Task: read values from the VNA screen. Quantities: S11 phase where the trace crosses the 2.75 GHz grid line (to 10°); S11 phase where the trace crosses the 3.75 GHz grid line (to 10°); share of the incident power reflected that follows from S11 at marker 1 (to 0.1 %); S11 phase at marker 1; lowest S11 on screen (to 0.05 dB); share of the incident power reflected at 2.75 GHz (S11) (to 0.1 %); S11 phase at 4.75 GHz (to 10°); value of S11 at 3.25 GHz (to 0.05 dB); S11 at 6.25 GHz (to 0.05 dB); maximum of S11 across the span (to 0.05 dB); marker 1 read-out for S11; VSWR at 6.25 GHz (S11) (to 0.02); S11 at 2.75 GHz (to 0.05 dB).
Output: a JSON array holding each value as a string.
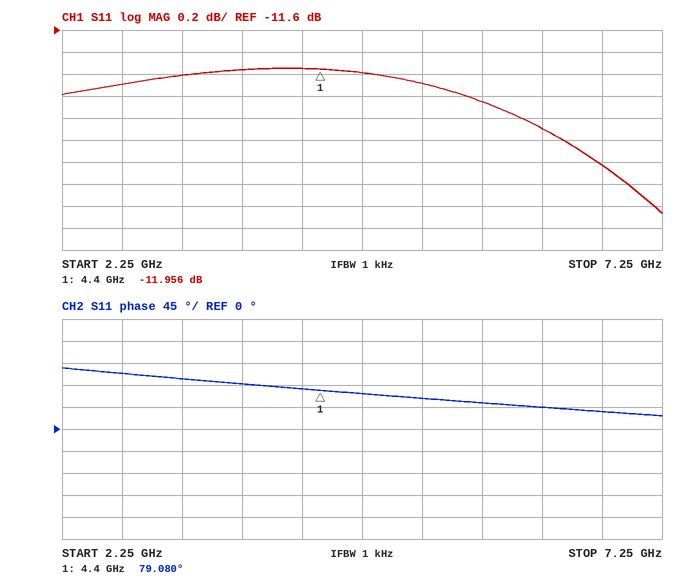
["110°", "90°", "6.4 %", "79.080°", "-13.25 dB", "6.2 %", "70°", "-12.00 dB", "-12.50 dB", "-11.95 dB", "-11.956 dB", "1.62", "-12.10 dB"]
